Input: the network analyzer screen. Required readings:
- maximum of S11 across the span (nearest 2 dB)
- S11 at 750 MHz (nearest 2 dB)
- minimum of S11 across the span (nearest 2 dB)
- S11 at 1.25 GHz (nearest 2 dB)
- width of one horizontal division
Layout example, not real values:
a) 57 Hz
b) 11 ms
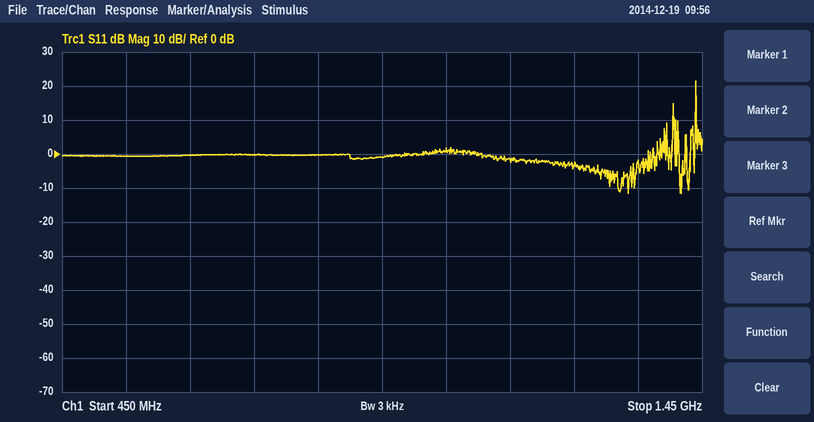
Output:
a) 22 dB
b) 0 dB
c) -12 dB
d) -4 dB
e) 100 MHz
